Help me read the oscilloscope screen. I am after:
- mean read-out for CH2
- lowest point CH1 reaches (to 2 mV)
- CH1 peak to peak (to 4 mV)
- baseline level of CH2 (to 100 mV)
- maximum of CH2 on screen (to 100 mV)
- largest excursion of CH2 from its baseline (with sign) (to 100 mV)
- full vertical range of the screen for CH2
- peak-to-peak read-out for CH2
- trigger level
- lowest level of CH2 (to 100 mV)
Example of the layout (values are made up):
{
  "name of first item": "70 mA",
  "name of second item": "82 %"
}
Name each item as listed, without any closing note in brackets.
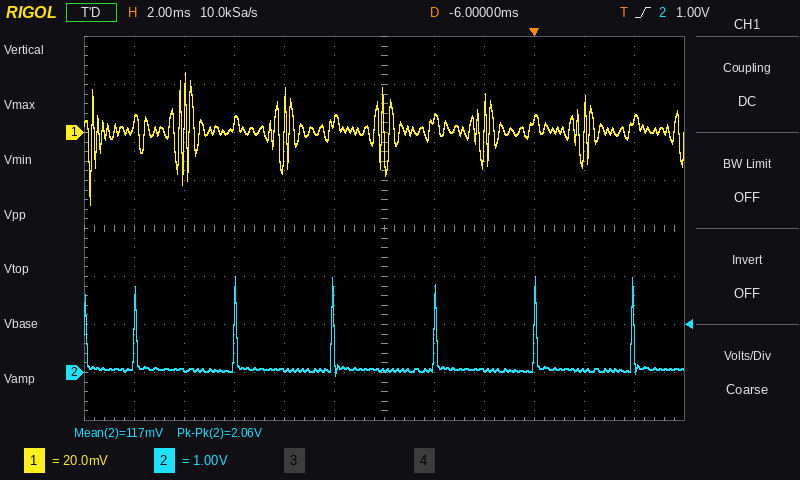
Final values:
{
  "mean read-out for CH2": "117 mV",
  "lowest point CH1 reaches": "-30 mV",
  "CH1 peak to peak": "56 mV",
  "baseline level of CH2": "100 mV",
  "maximum of CH2 on screen": "2.0 V",
  "largest excursion of CH2 from its baseline (with sign)": "+1.9 V",
  "full vertical range of the screen for CH2": "8 V",
  "peak-to-peak read-out for CH2": "2.06 V",
  "trigger level": "1.00 V",
  "lowest level of CH2": "-100 mV"
}
